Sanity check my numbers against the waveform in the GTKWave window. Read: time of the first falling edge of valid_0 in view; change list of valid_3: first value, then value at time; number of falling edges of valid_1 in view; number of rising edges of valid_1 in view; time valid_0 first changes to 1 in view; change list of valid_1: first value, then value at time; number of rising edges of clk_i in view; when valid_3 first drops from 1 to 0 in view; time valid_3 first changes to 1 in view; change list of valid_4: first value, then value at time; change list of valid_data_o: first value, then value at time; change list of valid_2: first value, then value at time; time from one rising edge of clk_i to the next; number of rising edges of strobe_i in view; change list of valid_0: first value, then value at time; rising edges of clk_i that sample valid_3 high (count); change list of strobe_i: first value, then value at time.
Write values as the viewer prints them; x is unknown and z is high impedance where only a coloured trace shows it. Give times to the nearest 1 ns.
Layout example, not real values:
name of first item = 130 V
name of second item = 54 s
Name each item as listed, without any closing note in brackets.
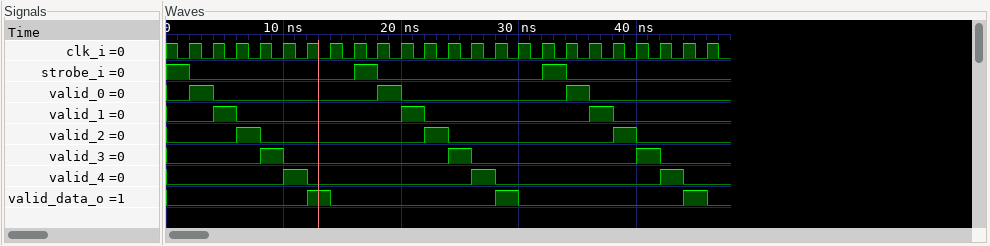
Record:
time of the first falling edge of valid_0 in view = 4 ns
change list of valid_3: first value, then value at time = 0, 1 at 8 ns, 0 at 10 ns, 1 at 24 ns, 0 at 26 ns, 1 at 40 ns, 0 at 42 ns
number of falling edges of valid_1 in view = 3
number of rising edges of valid_1 in view = 3
time valid_0 first changes to 1 in view = 2 ns
change list of valid_1: first value, then value at time = 0, 1 at 4 ns, 0 at 6 ns, 1 at 20 ns, 0 at 22 ns, 1 at 36 ns, 0 at 38 ns
number of rising edges of clk_i in view = 23
when valid_3 first drops from 1 to 0 in view = 10 ns
time valid_3 first changes to 1 in view = 8 ns
change list of valid_4: first value, then value at time = 0, 1 at 10 ns, 0 at 12 ns, 1 at 26 ns, 0 at 28 ns, 1 at 42 ns, 0 at 44 ns
change list of valid_data_o: first value, then value at time = 0, 1 at 12 ns, 0 at 14 ns, 1 at 28 ns, 0 at 30 ns, 1 at 44 ns, 0 at 46 ns
change list of valid_2: first value, then value at time = 0, 1 at 6 ns, 0 at 8 ns, 1 at 22 ns, 0 at 24 ns, 1 at 38 ns, 0 at 40 ns
time from one rising edge of clk_i to the next = 2 ns
number of rising edges of strobe_i in view = 2
change list of valid_0: first value, then value at time = 0, 1 at 2 ns, 0 at 4 ns, 1 at 18 ns, 0 at 20 ns, 1 at 34 ns, 0 at 36 ns
rising edges of clk_i that sample valid_3 high = 3
change list of strobe_i: first value, then value at time = 1, 0 at 2 ns, 1 at 16 ns, 0 at 18 ns, 1 at 32 ns, 0 at 34 ns
